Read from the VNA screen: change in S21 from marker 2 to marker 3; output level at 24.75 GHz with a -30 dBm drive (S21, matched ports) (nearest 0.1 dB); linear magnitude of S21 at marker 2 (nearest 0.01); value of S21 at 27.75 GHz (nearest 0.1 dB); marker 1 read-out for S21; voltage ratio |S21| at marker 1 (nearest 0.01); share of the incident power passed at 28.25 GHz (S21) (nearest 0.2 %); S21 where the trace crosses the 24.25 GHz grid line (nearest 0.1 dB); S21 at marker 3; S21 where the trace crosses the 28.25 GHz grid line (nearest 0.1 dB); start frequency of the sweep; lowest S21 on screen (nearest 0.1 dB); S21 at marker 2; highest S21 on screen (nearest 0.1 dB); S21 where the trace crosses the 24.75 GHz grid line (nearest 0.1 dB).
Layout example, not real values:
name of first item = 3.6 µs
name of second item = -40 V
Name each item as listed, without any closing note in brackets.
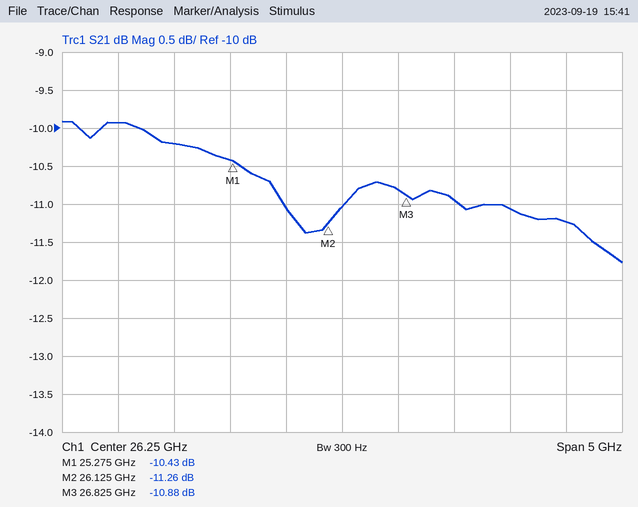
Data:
change in S21 from marker 2 to marker 3 = 0.38 dB
output level at 24.75 GHz with a -30 dBm drive (S21, matched ports) = -40.2 dBm
linear magnitude of S21 at marker 2 = 0.27
value of S21 at 27.75 GHz = -11.1 dB
marker 1 read-out for S21 = -10.43 dB
voltage ratio |S21| at marker 1 = 0.30
share of the incident power passed at 28.25 GHz (S21) = 7.6 %
S21 where the trace crosses the 24.25 GHz grid line = -9.9 dB
S21 at marker 3 = -10.88 dB
S21 where the trace crosses the 28.25 GHz grid line = -11.2 dB
start frequency of the sweep = 23.75 GHz
lowest S21 on screen = -11.8 dB
S21 at marker 2 = -11.26 dB
highest S21 on screen = -9.9 dB
S21 where the trace crosses the 24.75 GHz grid line = -10.2 dB
